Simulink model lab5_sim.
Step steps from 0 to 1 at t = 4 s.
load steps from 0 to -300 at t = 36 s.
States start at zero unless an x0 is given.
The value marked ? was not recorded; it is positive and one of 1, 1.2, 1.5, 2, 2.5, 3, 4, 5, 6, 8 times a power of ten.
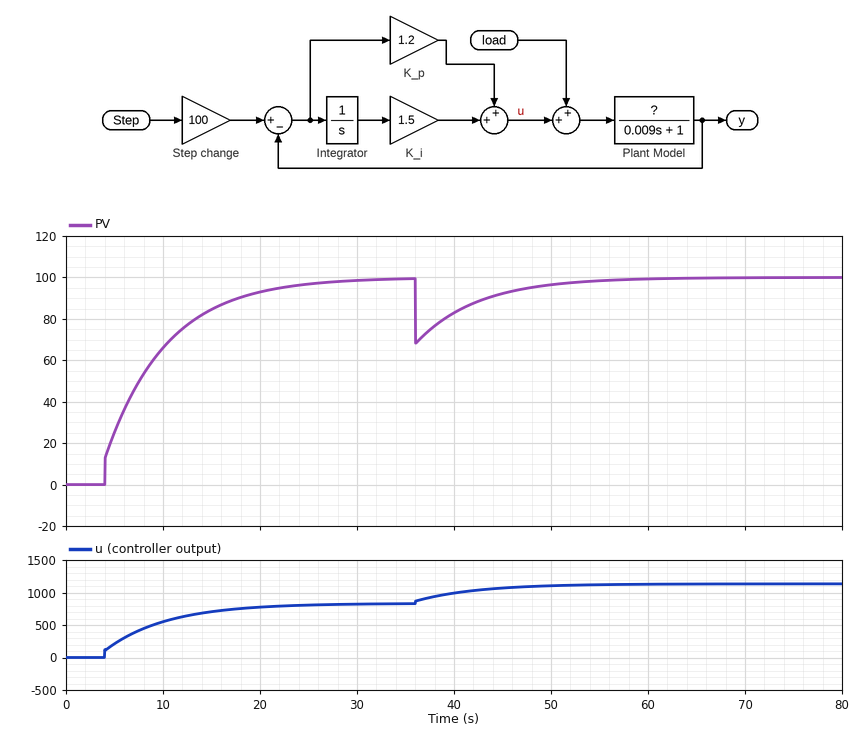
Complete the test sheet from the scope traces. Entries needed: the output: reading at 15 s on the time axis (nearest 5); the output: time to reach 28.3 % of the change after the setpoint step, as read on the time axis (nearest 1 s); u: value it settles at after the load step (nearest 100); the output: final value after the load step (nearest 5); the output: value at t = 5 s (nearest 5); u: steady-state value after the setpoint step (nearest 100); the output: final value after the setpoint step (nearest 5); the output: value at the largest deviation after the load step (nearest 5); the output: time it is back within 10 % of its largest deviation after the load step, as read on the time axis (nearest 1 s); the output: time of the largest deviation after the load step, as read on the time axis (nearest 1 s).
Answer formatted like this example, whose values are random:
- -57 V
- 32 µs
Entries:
- 85
- 5 s
- 1100
- 100
- 25
- 800
- 100
- 70
- 51 s
- 36 s
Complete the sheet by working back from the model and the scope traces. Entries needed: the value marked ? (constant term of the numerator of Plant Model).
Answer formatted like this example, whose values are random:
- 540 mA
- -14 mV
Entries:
- 0.12
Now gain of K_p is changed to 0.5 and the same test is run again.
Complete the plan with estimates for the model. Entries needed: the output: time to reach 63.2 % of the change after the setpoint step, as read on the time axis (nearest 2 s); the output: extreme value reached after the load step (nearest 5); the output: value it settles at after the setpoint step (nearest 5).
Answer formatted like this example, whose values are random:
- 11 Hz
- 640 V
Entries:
- 10 s
- 65
- 100
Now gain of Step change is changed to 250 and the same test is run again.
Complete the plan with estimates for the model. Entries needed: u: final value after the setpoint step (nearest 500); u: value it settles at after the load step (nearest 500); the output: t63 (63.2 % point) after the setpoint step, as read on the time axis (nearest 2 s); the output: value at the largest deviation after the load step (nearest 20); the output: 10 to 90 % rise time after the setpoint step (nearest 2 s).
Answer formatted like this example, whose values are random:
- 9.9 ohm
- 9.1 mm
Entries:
- 2000
- 2500
- 10 s
- 220
- 14 s
